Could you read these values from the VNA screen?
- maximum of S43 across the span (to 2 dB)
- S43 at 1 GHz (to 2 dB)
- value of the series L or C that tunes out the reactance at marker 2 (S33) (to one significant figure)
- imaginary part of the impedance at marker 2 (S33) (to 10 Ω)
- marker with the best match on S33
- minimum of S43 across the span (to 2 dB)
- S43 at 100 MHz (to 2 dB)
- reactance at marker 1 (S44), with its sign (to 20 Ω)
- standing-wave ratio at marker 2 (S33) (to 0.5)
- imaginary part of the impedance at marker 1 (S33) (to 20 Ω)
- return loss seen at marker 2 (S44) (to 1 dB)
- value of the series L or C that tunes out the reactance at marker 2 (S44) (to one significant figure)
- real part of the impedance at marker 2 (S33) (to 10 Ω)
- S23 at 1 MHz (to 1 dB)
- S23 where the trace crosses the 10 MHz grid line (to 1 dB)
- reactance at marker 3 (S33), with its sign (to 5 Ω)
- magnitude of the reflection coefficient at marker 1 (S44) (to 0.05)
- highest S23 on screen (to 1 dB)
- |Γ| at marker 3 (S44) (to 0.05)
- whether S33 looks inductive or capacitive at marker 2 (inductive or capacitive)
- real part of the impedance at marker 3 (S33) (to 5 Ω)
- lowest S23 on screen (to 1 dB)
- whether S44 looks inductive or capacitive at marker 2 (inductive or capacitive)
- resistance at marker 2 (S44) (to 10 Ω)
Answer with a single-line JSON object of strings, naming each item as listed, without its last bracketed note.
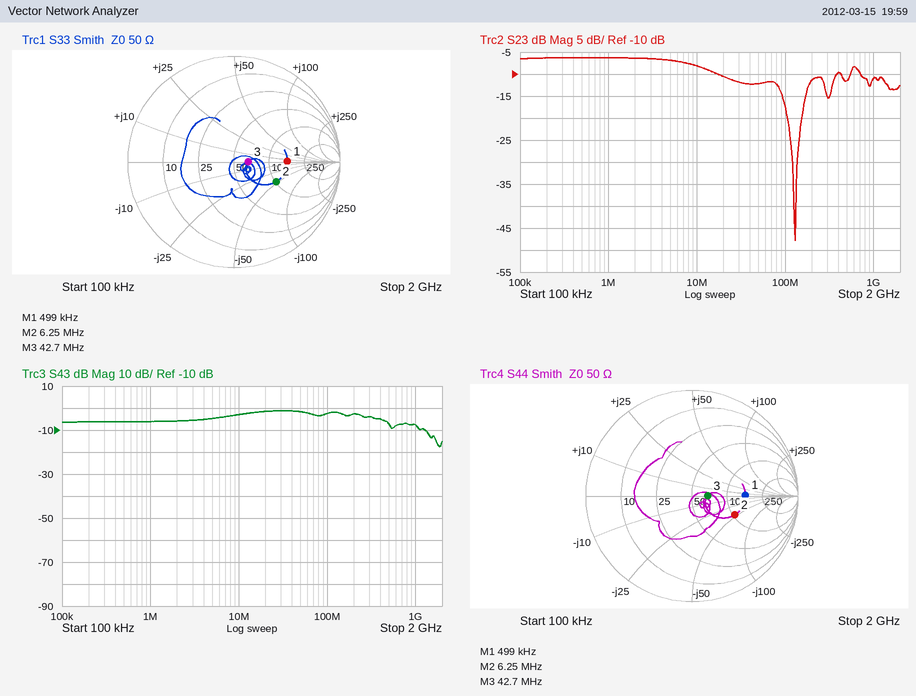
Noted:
{"maximum of S43 across the span": "-2 dB", "S43 at 1 GHz": "-8 dB", "value of the series L or C that tunes out the reactance at marker 2 (S33)": "1 µH", "imaginary part of the impedance at marker 2 (S33)": "-50 Ω", "marker with the best match on S33": "marker 3", "minimum of S43 across the span": "-18 dB", "S43 at 100 MHz": "-2 dB", "reactance at marker 1 (S44), with its sign": "0 Ω", "standing-wave ratio at marker 2 (S33)": "2.5", "imaginary part of the impedance at marker 1 (S33)": "0 Ω", "return loss seen at marker 2 (S44)": "7 dB", "value of the series L or C that tunes out the reactance at marker 2 (S44)": "1 µH", "real part of the impedance at marker 2 (S33)": "100 Ω", "S23 at 1 MHz": "-6 dB", "S23 where the trace crosses the 10 MHz grid line": "-8 dB", "reactance at marker 3 (S33), with its sign": "0 Ω", "magnitude of the reflection coefficient at marker 1 (S44)": "0.50", "highest S23 on screen": "-6 dB", "|Γ| at marker 3 (S44)": "0.15", "whether S33 looks inductive or capacitive at marker 2": "capacitive", "real part of the impedance at marker 3 (S33)": "65 Ω", "lowest S23 on screen": "-48 dB", "whether S44 looks inductive or capacitive at marker 2": "capacitive", "resistance at marker 2 (S44)": "100 Ω"}
